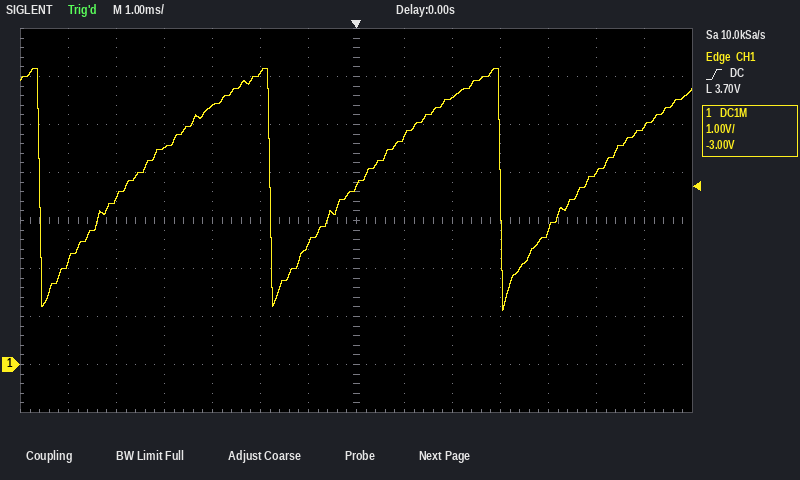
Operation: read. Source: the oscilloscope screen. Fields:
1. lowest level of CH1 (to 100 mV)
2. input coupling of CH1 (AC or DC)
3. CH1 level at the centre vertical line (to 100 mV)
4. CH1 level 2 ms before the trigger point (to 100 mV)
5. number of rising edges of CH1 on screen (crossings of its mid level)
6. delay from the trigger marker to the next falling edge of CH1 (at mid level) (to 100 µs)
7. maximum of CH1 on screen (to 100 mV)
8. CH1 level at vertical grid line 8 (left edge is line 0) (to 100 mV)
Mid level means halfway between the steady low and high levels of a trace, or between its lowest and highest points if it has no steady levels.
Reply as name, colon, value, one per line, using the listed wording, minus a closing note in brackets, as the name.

lowest level of CH1: 1.1 V
input coupling of CH1: DC
CH1 level at the centre vertical line: 3.7 V
CH1 level 2 ms before the trigger point: 6.1 V
number of rising edges of CH1 on screen: 3
delay from the trigger marker to the next falling edge of CH1 (at mid level): 3.0 ms
maximum of CH1 on screen: 6.2 V
CH1 level at vertical grid line 8 (left edge is line 0): 4.7 V
